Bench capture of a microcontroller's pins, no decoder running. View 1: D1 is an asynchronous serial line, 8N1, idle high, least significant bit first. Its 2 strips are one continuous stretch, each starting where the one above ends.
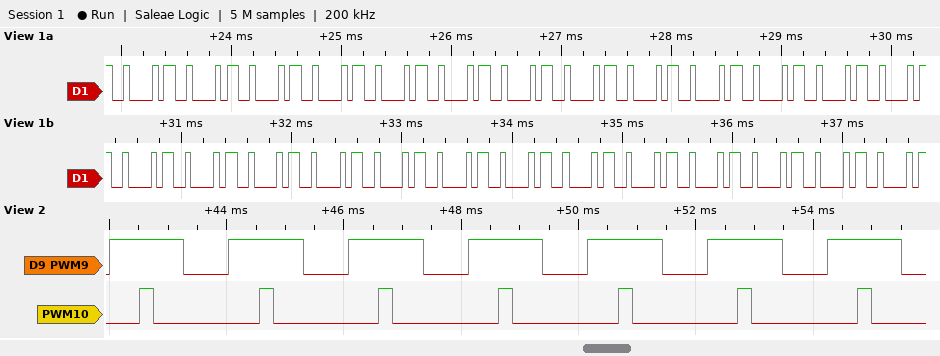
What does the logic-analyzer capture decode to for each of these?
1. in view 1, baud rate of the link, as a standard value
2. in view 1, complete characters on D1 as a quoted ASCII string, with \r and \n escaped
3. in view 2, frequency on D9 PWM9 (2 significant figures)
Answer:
19200 baud
"BBBBBBBBBBBBBBBBBBBBBBBBBB"
490 Hz
